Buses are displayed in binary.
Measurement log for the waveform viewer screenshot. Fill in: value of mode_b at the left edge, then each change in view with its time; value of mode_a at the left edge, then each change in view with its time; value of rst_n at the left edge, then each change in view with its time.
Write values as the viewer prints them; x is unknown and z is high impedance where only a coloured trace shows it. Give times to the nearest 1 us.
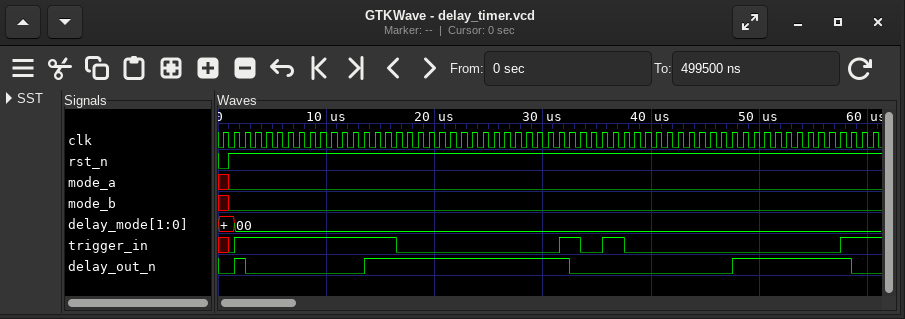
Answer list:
x, 0 at 1 us
x, 0 at 1 us
0, 1 at 1 us
